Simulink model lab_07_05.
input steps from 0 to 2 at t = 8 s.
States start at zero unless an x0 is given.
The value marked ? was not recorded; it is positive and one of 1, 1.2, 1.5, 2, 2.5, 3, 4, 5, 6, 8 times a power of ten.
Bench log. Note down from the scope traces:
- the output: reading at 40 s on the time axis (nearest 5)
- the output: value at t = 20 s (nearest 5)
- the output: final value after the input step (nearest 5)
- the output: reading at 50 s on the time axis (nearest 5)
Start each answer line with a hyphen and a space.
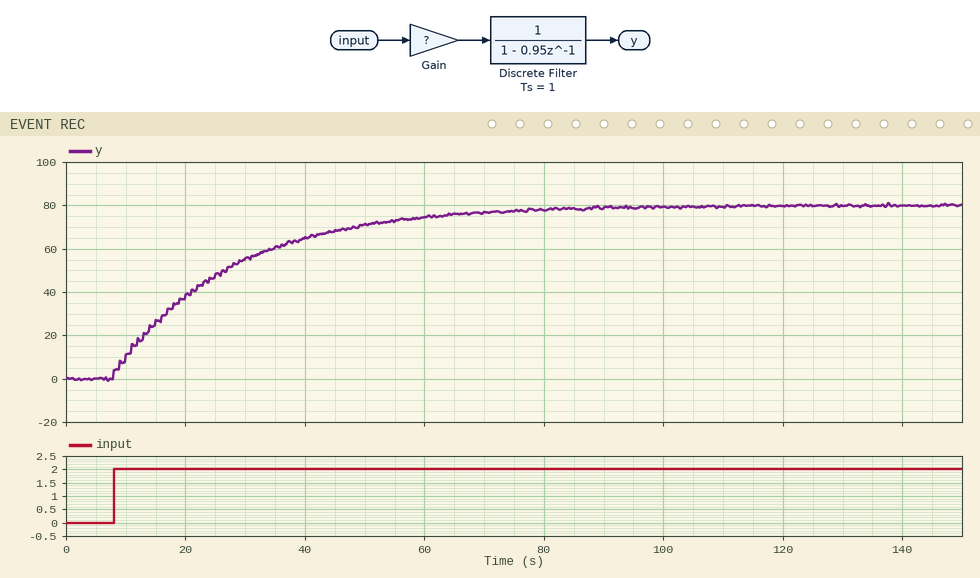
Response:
- 65
- 40
- 80
- 70
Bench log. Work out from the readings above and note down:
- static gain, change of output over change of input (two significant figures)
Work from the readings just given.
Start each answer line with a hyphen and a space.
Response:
- 40
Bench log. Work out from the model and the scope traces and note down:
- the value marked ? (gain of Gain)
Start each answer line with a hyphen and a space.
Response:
- 2
